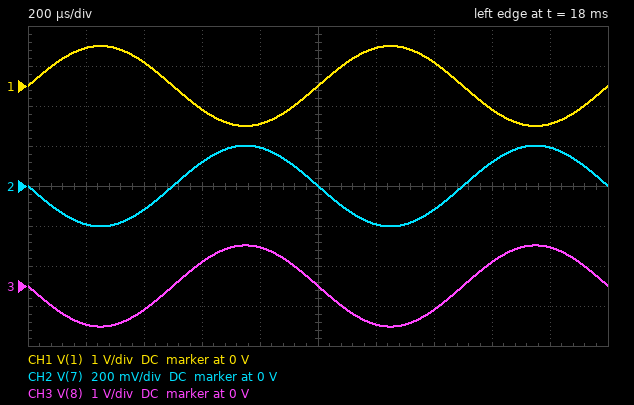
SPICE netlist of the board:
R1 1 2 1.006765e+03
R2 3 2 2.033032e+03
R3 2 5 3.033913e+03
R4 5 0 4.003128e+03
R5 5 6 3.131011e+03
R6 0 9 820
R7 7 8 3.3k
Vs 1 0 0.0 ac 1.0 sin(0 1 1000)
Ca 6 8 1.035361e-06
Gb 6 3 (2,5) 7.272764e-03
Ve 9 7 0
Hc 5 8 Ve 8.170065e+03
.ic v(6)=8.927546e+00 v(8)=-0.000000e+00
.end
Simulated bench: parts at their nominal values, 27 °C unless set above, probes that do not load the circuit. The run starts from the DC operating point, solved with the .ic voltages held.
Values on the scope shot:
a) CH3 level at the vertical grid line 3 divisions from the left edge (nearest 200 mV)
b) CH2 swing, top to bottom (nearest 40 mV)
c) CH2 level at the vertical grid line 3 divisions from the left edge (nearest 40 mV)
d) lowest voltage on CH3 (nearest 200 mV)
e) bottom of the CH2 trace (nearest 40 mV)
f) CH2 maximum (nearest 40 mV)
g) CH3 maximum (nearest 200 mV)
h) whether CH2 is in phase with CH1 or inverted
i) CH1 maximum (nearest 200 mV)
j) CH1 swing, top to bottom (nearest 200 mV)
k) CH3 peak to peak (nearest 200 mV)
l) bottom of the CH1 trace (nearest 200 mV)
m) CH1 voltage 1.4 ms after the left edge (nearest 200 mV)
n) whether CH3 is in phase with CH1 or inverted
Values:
600 mV
400 mV
120 mV
-1.0 V
-200 mV
200 mV
1.0 V
inverted
1.0 V
2.0 V
2.0 V
-1.0 V
600 mV
inverted
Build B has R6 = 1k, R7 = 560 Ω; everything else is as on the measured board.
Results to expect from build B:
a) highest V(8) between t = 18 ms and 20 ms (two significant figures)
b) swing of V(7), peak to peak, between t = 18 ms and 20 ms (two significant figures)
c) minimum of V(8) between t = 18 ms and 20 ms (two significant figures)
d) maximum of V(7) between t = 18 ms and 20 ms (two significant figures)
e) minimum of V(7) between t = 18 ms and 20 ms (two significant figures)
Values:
220 mV
280 mV
-220 mV
140 mV
-140 mV
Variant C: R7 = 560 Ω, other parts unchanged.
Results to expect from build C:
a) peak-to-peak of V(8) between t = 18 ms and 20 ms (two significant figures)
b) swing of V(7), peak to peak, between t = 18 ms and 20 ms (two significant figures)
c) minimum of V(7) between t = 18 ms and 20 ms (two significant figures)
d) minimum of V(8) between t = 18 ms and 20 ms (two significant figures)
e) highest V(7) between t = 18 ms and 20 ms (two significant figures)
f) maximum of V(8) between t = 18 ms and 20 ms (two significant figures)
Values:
370 mV
220 mV
-110 mV
-190 mV
110 mV
190 mV
